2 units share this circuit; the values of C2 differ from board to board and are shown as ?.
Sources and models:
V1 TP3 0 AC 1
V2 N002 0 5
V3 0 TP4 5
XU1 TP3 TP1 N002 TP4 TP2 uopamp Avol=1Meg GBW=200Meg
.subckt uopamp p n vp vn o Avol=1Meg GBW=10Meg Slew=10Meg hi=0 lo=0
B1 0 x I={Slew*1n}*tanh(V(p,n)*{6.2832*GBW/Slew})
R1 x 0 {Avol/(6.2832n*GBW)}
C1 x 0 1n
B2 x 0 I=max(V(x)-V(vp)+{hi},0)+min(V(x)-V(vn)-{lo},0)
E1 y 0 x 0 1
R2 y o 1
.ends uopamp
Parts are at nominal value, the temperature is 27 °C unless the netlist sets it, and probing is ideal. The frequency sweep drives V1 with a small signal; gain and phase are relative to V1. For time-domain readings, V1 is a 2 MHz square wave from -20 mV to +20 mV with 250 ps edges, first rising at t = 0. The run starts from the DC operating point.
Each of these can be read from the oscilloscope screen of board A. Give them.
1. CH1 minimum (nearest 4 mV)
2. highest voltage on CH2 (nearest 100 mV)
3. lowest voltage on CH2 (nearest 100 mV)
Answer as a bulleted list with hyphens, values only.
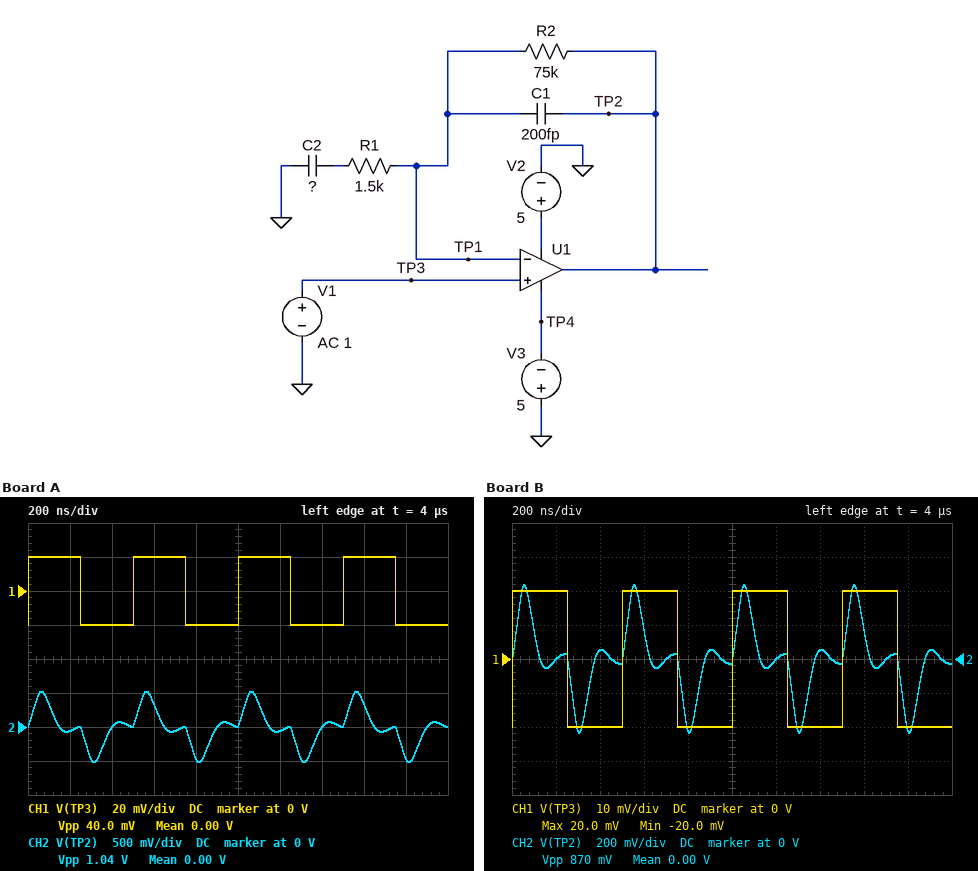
- -20 mV
- 500 mV
- -500 mV
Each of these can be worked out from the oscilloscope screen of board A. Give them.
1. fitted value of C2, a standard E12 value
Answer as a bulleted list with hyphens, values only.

- 12 pF
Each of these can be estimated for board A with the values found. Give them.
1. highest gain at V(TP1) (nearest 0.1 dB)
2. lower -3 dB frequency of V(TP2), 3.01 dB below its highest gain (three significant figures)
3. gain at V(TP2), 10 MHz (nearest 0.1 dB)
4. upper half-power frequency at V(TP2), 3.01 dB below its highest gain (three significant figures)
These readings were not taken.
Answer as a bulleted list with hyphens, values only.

- 2.1 dB
- 3.02 MHz
- 24.1 dB
- 8.34 MHz
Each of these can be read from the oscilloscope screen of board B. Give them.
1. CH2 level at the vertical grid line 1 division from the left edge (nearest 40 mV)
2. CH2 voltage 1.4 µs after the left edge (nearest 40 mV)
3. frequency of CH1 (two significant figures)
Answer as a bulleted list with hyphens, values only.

- 0 V
- 40 mV
- 2.0 MHz
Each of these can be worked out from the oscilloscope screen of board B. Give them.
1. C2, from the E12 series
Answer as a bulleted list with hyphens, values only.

- 8.2 pF
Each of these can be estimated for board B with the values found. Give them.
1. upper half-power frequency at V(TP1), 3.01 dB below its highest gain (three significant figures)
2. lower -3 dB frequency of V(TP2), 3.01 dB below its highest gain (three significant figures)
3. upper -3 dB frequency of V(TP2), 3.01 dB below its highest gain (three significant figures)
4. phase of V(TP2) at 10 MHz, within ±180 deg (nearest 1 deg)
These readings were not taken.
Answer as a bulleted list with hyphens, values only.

- 8.21 MHz
- 3.64 MHz
- 10.1 MHz
- -46 deg
